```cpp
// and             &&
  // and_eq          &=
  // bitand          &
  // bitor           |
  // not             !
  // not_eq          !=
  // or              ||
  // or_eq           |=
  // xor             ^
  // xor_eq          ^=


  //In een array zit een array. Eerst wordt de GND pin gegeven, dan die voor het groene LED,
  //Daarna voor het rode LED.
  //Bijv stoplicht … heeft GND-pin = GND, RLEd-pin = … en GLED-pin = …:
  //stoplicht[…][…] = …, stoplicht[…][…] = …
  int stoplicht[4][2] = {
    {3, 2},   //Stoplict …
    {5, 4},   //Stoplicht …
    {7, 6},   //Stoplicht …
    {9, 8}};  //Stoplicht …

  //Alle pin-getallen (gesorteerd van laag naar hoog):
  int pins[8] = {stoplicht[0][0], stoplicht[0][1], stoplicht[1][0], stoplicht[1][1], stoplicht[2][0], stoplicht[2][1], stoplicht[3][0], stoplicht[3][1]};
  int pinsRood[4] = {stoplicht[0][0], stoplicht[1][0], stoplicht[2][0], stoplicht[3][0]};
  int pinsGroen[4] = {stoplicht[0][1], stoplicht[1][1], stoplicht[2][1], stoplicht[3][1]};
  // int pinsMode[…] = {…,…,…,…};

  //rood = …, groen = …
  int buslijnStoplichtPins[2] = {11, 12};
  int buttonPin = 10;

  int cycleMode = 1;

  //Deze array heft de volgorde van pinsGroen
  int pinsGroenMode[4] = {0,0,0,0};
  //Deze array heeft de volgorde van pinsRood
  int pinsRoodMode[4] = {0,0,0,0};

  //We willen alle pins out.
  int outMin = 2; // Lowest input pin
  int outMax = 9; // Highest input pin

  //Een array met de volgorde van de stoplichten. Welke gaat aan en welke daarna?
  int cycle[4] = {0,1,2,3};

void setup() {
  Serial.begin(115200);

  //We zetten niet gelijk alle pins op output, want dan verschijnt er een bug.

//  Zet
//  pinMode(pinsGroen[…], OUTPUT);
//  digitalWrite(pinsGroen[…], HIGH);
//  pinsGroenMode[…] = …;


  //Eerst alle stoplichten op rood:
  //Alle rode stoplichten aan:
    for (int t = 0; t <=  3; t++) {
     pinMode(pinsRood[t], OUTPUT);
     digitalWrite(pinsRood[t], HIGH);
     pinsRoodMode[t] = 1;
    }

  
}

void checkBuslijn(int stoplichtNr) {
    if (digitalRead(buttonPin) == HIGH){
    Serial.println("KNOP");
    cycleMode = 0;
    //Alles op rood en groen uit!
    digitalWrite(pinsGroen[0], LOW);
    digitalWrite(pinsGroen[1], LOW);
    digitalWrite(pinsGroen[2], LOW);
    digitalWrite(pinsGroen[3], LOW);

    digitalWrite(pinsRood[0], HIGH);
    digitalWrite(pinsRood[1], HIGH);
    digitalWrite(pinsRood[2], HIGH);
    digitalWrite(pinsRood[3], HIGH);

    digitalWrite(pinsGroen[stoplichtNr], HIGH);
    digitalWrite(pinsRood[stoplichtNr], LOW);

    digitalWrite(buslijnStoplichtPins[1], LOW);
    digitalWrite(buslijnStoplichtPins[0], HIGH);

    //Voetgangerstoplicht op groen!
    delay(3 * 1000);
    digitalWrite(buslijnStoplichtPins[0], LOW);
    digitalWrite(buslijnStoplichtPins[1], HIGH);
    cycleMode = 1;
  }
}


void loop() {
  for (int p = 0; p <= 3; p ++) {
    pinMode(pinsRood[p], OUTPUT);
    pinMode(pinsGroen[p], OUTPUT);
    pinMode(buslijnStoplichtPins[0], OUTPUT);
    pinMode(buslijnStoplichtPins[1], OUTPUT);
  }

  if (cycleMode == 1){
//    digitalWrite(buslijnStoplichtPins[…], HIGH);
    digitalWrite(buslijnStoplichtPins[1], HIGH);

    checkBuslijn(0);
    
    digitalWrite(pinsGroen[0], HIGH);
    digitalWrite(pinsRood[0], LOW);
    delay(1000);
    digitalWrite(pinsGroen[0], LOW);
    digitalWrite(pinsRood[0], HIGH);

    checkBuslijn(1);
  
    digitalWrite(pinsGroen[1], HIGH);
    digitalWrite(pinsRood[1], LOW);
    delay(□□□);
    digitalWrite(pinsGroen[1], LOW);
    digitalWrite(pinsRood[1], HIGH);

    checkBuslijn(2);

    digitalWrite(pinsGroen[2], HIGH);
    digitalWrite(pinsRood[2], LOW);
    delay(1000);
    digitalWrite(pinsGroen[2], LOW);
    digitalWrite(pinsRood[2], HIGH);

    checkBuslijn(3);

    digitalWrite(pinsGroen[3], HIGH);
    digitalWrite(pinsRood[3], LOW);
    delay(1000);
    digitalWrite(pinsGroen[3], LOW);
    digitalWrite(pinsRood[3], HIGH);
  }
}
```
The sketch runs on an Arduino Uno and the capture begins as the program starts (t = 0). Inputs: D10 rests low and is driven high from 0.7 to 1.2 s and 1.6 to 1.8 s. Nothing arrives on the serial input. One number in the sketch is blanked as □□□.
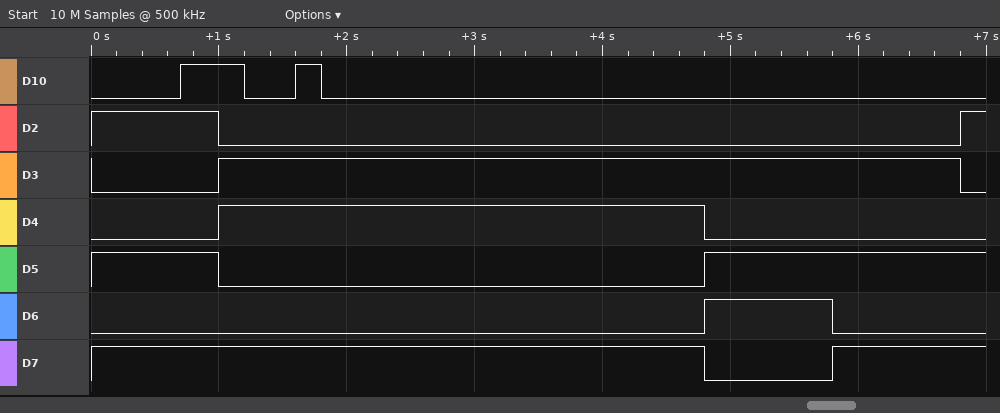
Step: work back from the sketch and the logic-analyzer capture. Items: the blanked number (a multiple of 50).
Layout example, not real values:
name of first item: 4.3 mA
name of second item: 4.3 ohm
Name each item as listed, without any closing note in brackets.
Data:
the blanked number: 800
